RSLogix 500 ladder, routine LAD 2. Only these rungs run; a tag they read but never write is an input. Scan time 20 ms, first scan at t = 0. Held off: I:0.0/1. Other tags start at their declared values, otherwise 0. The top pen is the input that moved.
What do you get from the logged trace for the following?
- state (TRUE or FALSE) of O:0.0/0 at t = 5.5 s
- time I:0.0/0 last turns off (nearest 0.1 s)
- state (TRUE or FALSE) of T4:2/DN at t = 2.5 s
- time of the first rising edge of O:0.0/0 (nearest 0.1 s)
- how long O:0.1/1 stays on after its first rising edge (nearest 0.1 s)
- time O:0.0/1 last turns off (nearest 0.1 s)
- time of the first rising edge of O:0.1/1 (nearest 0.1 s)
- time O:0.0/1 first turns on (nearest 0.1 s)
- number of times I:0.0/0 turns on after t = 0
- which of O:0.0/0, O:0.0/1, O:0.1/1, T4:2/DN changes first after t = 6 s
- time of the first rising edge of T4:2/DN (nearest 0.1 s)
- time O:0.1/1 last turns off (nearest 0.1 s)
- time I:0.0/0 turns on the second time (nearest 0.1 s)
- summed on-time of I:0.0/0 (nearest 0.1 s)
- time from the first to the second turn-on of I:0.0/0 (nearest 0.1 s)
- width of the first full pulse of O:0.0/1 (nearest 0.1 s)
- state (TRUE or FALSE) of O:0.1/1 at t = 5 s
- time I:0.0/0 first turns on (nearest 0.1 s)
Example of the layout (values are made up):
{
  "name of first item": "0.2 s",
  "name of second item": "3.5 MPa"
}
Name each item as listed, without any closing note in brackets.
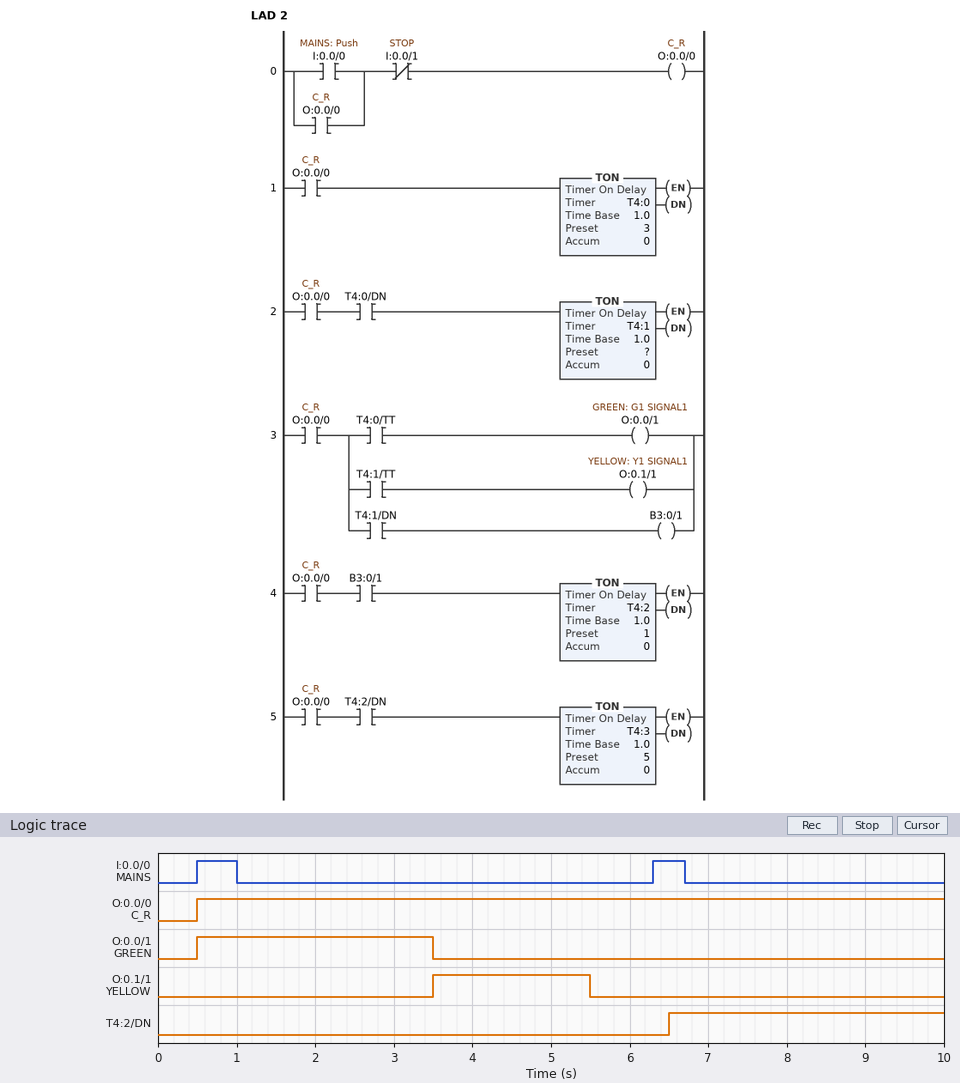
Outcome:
{
  "state (TRUE or FALSE) of O:0.0/0 at t = 5.5 s": "TRUE",
  "time I:0.0/0 last turns off": "6.7 s",
  "state (TRUE or FALSE) of T4:2/DN at t = 2.5 s": "FALSE",
  "time of the first rising edge of O:0.0/0": "0.5 s",
  "how long O:0.1/1 stays on after its first rising edge": "2.0 s",
  "time O:0.0/1 last turns off": "3.5 s",
  "time of the first rising edge of O:0.1/1": "3.5 s",
  "time O:0.0/1 first turns on": "0.5 s",
  "number of times I:0.0/0 turns on after t = 0": "2",
  "which of O:0.0/0, O:0.0/1, O:0.1/1, T4:2/DN changes first after t = 6 s": "T4:2/DN",
  "time of the first rising edge of T4:2/DN": "6.5 s",
  "time O:0.1/1 last turns off": "5.5 s",
  "time I:0.0/0 turns on the second time": "6.3 s",
  "summed on-time of I:0.0/0": "0.9 s",
  "time from the first to the second turn-on of I:0.0/0": "5.8 s",
  "width of the first full pulse of O:0.0/1": "3.0 s",
  "state (TRUE or FALSE) of O:0.1/1 at t = 5 s": "TRUE",
  "time I:0.0/0 first turns on": "0.5 s"
}
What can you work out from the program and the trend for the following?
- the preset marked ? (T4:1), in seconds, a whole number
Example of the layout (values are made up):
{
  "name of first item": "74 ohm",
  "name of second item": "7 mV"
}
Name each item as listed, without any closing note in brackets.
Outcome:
{
  "the preset marked ? (T4:1), in seconds, a whole number": "2 s"
}
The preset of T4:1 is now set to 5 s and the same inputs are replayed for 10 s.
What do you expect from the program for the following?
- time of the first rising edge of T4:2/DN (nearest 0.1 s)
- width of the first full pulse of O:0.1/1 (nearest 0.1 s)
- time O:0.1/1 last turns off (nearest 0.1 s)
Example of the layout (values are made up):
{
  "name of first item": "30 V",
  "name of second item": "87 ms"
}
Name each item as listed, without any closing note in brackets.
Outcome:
{
  "time of the first rising edge of T4:2/DN": "9.5 s",
  "width of the first full pulse of O:0.1/1": "5.0 s",
  "time O:0.1/1 last turns off": "8.5 s"
}
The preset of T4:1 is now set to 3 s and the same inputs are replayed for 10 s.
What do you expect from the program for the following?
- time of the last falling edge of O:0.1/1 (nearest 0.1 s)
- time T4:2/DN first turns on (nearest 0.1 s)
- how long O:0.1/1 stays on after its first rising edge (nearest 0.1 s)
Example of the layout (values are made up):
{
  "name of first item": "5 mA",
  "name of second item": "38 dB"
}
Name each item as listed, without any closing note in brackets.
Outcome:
{
  "time of the last falling edge of O:0.1/1": "6.5 s",
  "time T4:2/DN first turns on": "7.5 s",
  "how long O:0.1/1 stays on after its first rising edge": "3.0 s"
}
